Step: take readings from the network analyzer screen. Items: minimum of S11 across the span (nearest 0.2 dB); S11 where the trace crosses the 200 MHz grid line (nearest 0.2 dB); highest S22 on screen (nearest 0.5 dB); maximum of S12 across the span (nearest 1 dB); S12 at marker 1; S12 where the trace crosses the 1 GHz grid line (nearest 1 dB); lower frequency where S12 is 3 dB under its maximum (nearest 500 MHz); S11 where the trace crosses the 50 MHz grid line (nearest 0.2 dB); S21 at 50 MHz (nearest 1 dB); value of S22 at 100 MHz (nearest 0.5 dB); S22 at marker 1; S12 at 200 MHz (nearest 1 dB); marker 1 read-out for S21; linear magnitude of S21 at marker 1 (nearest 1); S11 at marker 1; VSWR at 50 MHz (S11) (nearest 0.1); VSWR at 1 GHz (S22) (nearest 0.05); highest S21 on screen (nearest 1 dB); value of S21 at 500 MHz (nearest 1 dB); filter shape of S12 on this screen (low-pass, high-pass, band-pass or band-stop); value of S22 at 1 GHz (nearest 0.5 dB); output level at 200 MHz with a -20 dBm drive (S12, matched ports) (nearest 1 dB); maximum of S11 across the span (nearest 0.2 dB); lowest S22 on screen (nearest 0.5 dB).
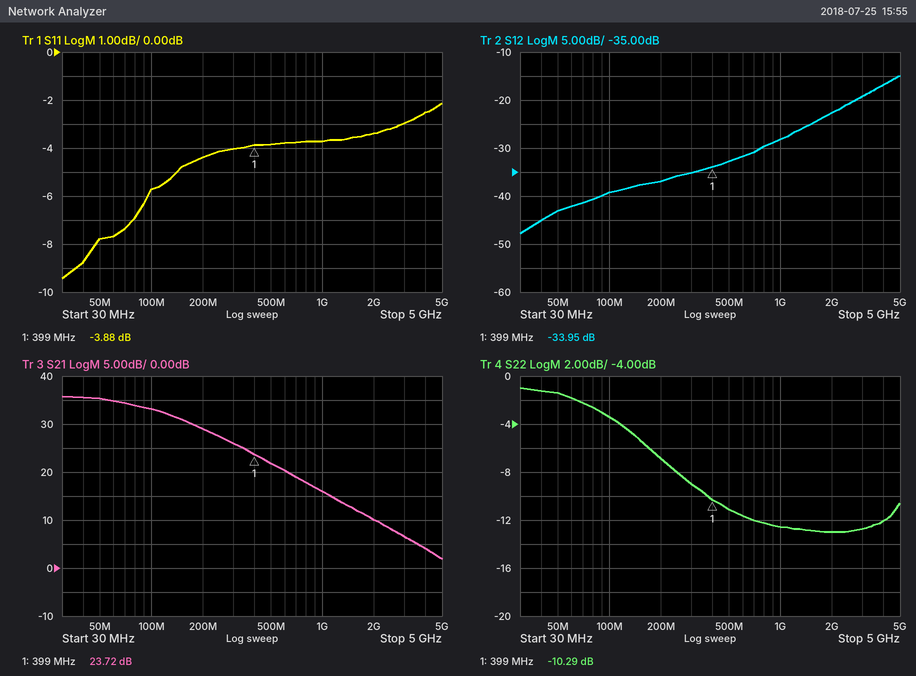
-9.4 dB
-4.4 dB
-1.0 dB
-15 dB
-33.95 dB
-28 dB
3.5 GHz
-7.8 dB
35 dB
-3.5 dB
-10.29 dB
-37 dB
23.72 dB
15
-3.88 dB
2.4
1.60
36 dB
22 dB
high-pass
-12.5 dB
-57 dBm
-2.2 dB
-13.0 dB
